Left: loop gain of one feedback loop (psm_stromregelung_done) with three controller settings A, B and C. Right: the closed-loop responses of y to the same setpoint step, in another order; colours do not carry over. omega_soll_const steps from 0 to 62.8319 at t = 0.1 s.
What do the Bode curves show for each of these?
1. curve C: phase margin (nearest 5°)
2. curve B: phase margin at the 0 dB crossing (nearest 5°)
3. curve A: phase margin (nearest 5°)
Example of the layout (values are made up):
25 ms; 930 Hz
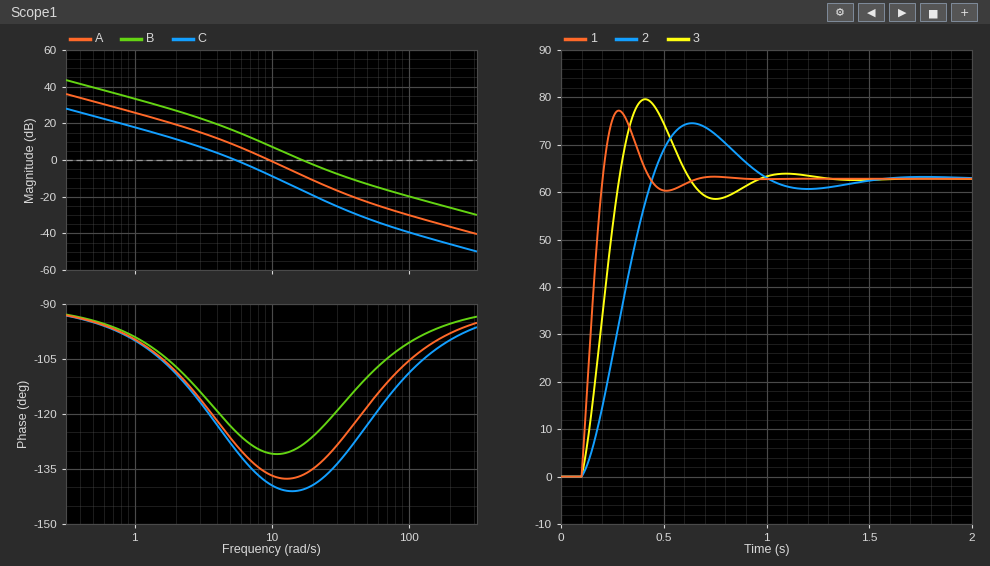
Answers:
50°; 50°; 45°
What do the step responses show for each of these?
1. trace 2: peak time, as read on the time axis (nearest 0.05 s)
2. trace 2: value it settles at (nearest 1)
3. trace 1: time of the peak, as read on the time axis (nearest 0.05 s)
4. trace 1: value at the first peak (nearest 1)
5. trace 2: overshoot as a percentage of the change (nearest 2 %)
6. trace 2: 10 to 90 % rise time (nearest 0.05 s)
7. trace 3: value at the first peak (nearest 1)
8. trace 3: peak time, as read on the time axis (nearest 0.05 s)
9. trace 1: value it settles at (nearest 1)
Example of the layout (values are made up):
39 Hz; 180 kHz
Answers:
0.65 s; 63; 0.30 s; 77; 18 %; 0.25 s; 80; 0.40 s; 63
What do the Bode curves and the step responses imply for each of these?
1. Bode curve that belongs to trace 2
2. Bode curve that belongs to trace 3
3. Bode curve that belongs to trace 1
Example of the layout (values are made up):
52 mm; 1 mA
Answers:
C; A; B
